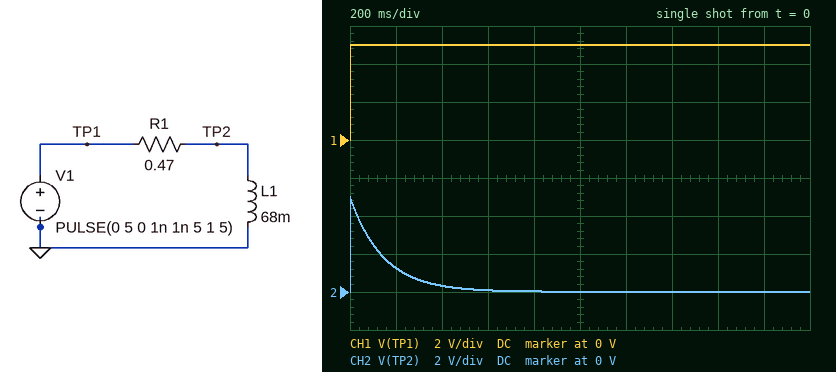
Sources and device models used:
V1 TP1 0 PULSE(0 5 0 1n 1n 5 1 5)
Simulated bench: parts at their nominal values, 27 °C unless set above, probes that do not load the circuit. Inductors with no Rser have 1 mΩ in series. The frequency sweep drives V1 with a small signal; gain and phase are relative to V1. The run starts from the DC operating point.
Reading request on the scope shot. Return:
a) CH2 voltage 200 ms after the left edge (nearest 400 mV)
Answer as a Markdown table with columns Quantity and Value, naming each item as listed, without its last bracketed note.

| Quantity | Value |
|---|---|
| CH2 voltage 200 ms after the left edge | 1.2 V |
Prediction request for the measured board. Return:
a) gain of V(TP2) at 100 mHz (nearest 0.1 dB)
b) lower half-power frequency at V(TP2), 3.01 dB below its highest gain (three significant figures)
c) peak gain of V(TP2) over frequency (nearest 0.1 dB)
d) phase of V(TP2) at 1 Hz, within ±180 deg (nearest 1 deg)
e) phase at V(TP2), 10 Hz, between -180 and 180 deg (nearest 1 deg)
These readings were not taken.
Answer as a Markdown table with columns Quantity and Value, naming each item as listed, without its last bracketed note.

| Quantity | Value |
|---|---|
| gain of V(TP2) at 100 mHz | -20.9 dB |
| lower half-power frequency at V(TP2), 3.01 dB below its highest gain | 1.10 Hz |
| peak gain of V(TP2) over frequency | 0 dB |
| phase of V(TP2) at 1 Hz, within ±180 deg | 48 deg |
| phase at V(TP2), 10 Hz, between -180 and 180 deg | 6 deg |
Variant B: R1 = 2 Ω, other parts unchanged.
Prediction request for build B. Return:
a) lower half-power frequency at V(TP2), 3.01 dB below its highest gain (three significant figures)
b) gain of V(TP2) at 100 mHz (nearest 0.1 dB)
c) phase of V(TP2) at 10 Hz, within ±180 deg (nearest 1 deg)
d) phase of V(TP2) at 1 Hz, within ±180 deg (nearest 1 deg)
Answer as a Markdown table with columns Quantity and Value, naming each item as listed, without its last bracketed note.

| Quantity | Value |
|---|---|
| lower half-power frequency at V(TP2), 3.01 dB below its highest gain | 4.68 Hz |
| gain of V(TP2) at 100 mHz | -33.4 dB |
| phase of V(TP2) at 10 Hz, within ±180 deg | 25 deg |
| phase of V(TP2) at 1 Hz, within ±180 deg | 78 deg |
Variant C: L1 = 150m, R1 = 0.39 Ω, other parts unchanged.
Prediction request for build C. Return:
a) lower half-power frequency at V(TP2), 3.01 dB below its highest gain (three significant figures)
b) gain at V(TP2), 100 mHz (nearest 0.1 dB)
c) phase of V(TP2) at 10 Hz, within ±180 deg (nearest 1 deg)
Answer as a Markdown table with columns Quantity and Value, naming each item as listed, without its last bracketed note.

| Quantity | Value |
|---|---|
| lower half-power frequency at V(TP2), 3.01 dB below its highest gain | 415 mHz |
| gain at V(TP2), 100 mHz | -12.6 dB |
| phase of V(TP2) at 10 Hz, within ±180 deg | 2 deg |
